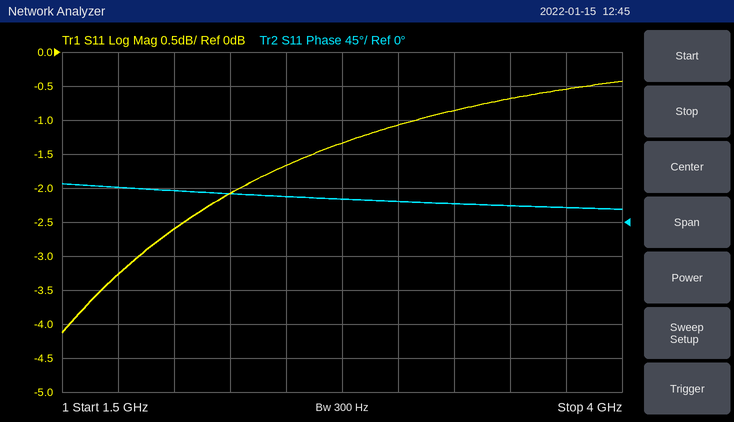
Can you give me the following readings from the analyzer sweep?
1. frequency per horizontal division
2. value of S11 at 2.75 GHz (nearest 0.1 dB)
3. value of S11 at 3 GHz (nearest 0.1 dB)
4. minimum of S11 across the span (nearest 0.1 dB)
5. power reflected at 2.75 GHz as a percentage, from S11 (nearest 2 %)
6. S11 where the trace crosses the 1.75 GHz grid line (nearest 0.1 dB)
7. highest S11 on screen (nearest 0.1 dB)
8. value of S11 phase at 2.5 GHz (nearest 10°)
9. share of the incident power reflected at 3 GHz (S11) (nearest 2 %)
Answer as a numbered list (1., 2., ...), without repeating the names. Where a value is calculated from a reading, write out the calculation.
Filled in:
1. 250 MHz
2. -1.3 dB
3. -1.1 dB
4. -4.1 dB
5. 10^(-1.3/10) ≈ 74 %
6. -3.3 dB
7. -0.4 dB
8. 30°
9. 10^(-1.1/10) ≈ 78 %
